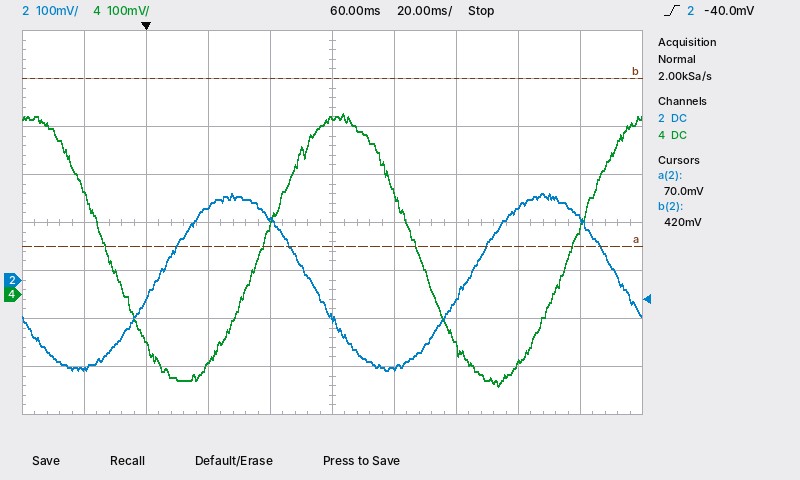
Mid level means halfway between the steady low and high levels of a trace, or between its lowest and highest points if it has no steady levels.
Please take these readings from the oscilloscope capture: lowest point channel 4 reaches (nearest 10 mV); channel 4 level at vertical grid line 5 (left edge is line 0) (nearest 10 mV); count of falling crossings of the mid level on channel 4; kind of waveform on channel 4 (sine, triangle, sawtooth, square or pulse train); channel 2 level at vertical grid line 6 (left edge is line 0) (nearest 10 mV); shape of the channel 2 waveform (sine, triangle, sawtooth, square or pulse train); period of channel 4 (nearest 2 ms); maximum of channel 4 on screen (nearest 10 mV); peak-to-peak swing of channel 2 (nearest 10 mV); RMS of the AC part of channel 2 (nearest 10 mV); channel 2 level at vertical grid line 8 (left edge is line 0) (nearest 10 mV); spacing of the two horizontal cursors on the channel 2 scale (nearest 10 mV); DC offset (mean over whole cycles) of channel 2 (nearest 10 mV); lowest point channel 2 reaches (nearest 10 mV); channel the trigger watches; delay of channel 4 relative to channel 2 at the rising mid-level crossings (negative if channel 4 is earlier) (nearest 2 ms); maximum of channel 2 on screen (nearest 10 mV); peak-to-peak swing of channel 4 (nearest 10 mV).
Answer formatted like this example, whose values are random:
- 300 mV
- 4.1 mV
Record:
- -190 mV
- 370 mV
- 2
- sine
- -180 mV
- sine
- 100 ms
- 380 mV
- 370 mV
- 130 mV
- 150 mV
- 350 mV
- 0 mV
- -190 mV
- channel 2
- +34 ms
- 180 mV
- 570 mV
